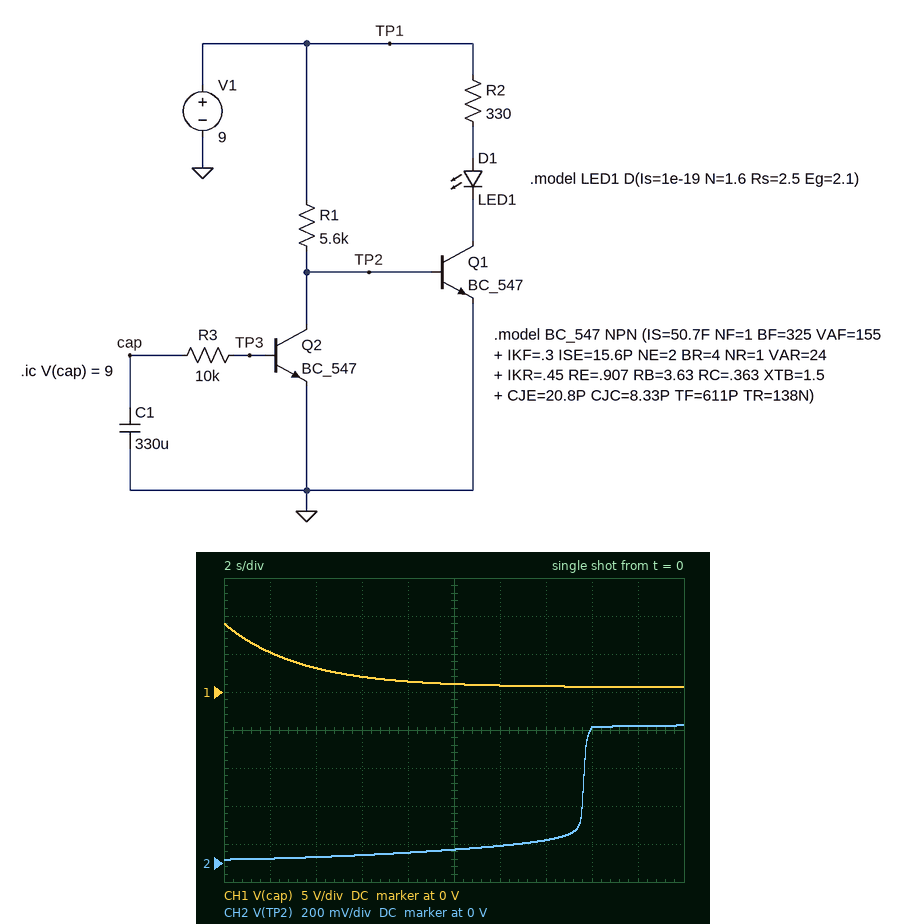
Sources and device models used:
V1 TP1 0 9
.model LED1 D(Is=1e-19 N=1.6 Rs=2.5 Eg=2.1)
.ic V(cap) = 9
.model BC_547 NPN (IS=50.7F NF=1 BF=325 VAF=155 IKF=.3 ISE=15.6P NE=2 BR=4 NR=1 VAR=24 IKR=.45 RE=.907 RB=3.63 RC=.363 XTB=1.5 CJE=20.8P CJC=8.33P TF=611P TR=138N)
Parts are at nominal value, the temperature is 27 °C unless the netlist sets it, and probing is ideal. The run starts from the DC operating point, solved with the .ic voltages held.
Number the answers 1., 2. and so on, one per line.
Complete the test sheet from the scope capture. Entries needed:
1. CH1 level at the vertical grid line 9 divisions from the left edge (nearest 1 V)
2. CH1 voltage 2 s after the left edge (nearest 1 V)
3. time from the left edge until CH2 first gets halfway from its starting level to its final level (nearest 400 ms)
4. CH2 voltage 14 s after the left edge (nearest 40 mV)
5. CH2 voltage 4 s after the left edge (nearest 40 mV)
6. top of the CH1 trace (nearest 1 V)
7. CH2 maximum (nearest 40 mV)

1. 1 V
2. 5 V
3. 15.6 s
4. 120 mV
5. 40 mV
6. 9 V
7. 720 mV
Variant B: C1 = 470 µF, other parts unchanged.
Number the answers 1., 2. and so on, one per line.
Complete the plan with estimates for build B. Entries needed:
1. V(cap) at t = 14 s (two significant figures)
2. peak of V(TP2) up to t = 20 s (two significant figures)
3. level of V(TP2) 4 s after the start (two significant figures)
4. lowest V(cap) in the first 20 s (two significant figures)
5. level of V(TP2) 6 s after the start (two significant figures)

1. 1.1 V
2. 120 mV
3. 26 mV
4. 750 mV
5. 32 mV
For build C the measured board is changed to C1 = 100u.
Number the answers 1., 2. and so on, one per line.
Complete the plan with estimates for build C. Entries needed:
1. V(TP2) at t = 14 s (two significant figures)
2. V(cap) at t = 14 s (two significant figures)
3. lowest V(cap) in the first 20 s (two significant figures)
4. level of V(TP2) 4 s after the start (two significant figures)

1. 730 mV
2. 530 mV
3. 510 mV
4. 110 mV
